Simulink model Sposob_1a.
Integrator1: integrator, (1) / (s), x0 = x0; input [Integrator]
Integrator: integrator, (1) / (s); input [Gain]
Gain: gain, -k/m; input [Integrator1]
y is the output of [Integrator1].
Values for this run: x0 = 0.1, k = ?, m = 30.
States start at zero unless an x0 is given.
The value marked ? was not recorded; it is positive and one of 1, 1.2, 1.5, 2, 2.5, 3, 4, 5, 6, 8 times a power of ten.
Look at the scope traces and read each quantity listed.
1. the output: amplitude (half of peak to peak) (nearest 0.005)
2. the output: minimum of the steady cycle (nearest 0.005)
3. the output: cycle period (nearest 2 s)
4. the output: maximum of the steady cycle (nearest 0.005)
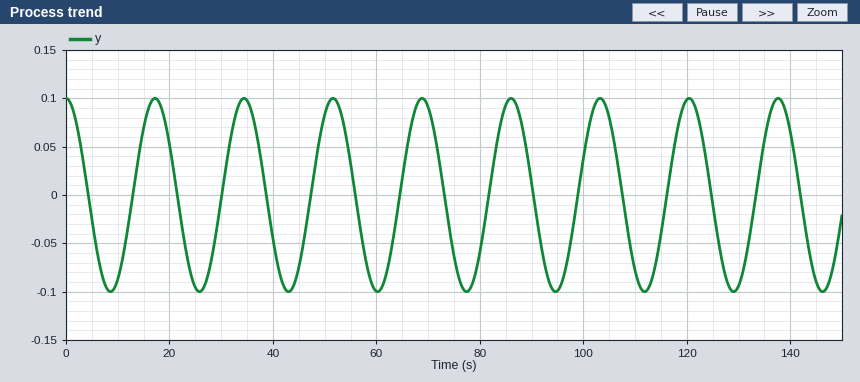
0.100
-0.100
18 s
0.100
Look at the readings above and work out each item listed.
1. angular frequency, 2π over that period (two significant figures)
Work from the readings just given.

0.35 rad/s
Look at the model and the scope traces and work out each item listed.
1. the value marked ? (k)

4
